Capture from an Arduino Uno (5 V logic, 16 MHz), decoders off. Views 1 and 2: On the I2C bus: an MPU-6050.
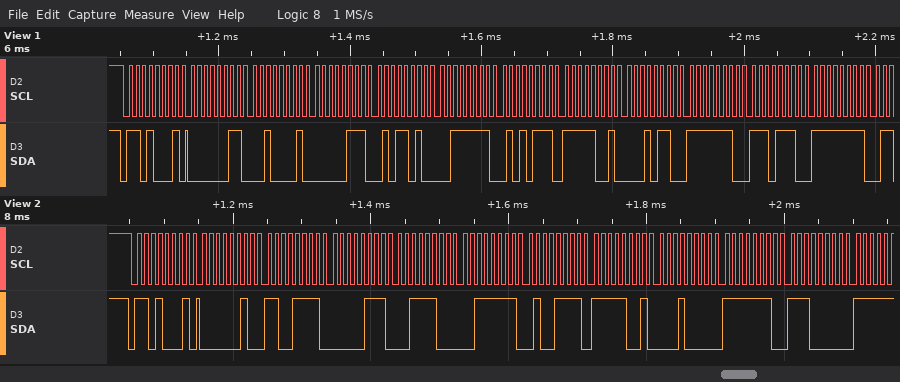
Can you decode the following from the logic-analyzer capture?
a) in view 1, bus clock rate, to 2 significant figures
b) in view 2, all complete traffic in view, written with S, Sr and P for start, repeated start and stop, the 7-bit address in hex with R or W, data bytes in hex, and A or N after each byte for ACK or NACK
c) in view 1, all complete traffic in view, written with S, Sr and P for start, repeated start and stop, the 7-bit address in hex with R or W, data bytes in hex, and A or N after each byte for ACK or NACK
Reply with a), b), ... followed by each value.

a) 100 kHz
b) S 68R A 02 A CF A 07 A 3C A 3F A 4F A F9 A 10 A FE A E0 A
c) S 68R A 03 A 21 A 07 A 5A A 3F A 57 A F9 A 16 A FE A EE A FF A
